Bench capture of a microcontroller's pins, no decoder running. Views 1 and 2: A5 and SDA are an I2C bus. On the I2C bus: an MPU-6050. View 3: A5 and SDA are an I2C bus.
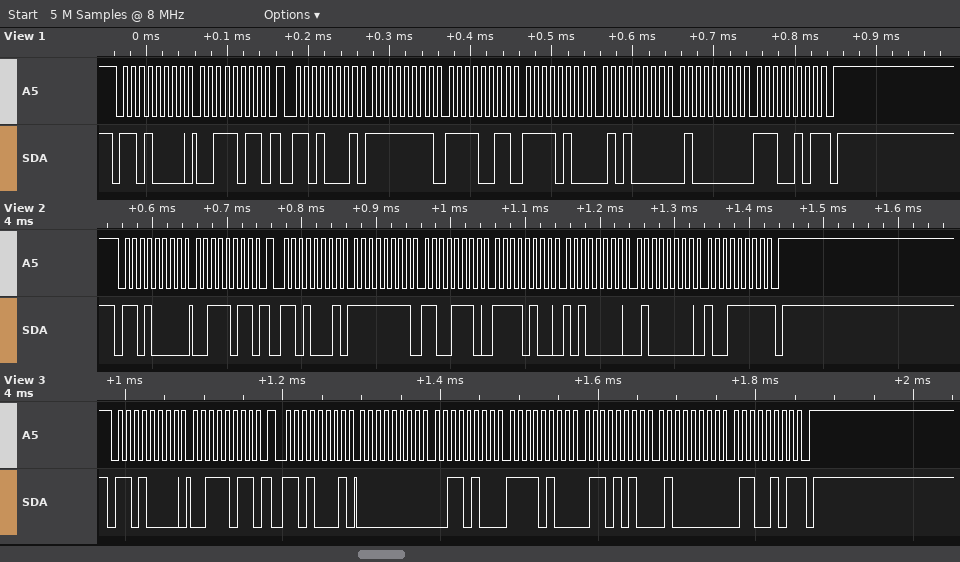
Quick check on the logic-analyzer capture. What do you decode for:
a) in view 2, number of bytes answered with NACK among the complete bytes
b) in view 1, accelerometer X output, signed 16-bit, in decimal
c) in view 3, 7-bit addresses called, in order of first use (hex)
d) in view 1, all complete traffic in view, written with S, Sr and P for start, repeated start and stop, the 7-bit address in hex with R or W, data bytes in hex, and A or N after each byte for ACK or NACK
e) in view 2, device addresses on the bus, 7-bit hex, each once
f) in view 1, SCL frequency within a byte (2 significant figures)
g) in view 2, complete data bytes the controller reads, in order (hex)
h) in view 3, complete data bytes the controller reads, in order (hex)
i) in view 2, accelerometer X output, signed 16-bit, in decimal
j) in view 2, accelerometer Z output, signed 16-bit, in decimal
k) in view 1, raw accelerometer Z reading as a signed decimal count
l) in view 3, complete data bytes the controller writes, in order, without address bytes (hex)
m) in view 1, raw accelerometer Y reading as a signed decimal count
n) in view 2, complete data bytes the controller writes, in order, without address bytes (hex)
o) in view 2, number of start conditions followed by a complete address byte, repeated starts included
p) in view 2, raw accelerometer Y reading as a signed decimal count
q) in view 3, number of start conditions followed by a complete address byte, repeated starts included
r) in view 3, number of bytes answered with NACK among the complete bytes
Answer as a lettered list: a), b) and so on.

a) 1
b) -13
c) 0x68
d) S 68W A 3B A Sr 68R A FF A F3 A F4 A 50 A 40 A E5 N P
e) 0x68
f) 100 kHz
g) FF CE F4 A0 40 9F
h) 00 34 F4 6A 40 65
i) -50
j) 16543
k) 16613
l) 3B
m) -2992
n) 3B
o) 2
p) -2912
q) 2
r) 1
